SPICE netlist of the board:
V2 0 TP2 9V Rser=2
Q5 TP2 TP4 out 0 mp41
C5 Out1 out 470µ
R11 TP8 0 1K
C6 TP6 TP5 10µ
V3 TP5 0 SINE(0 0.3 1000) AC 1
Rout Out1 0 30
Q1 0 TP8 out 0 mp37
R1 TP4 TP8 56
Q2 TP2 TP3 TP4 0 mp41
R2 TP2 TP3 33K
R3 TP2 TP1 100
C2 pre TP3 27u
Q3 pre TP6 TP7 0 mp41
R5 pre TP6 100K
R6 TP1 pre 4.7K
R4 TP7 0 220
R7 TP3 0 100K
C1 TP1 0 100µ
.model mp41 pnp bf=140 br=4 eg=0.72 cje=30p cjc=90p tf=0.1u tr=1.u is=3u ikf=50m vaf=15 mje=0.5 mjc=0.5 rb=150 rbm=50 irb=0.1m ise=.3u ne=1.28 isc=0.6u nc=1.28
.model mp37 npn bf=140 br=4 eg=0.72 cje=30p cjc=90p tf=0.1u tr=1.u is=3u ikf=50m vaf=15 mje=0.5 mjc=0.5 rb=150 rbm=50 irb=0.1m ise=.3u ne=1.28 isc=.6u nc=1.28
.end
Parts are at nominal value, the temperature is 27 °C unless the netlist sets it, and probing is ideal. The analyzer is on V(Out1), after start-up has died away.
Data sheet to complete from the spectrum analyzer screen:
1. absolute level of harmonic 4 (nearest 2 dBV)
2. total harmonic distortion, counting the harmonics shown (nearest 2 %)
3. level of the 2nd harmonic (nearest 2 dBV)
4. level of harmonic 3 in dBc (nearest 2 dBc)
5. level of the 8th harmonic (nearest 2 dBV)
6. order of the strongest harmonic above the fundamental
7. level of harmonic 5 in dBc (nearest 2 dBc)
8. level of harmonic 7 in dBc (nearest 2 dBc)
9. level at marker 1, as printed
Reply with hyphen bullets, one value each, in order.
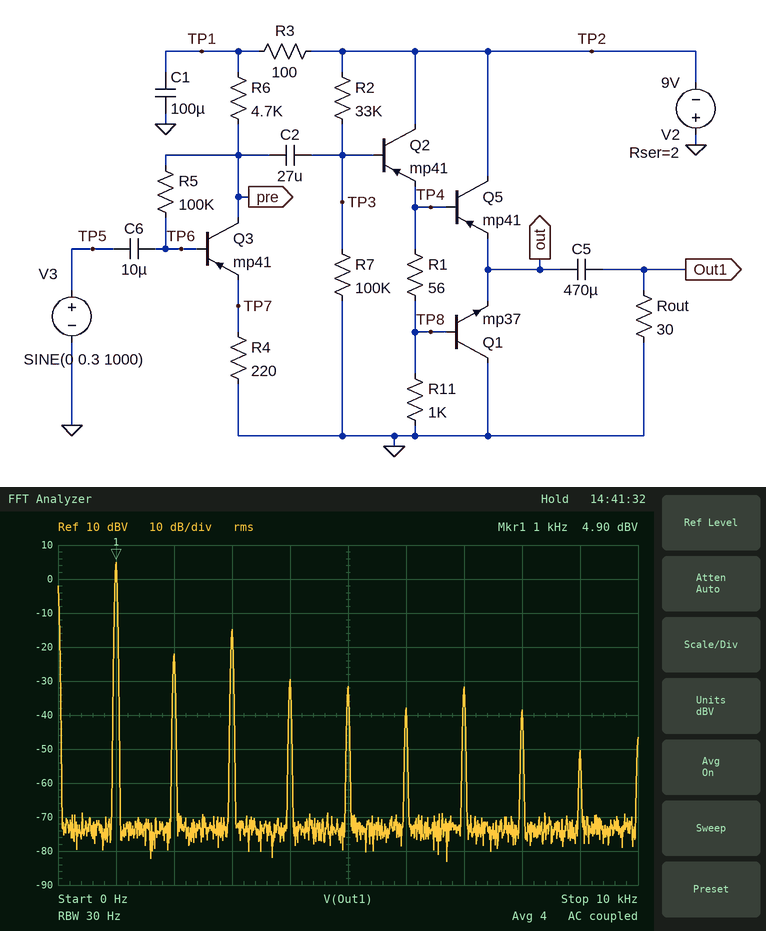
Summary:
- -30 dBV
- 12 %
- -22 dBV
- -20 dBc
- -38 dBV
- 3
- -36 dBc
- -36 dBc
- 4.90 dBV
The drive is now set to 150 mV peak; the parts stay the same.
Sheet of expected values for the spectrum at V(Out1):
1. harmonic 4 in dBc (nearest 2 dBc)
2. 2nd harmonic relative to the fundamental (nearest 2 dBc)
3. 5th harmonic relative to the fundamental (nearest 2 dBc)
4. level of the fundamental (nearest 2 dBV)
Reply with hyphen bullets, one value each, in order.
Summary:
- -52 dBc
- -48 dBc
- -40 dBc
- 0 dBV
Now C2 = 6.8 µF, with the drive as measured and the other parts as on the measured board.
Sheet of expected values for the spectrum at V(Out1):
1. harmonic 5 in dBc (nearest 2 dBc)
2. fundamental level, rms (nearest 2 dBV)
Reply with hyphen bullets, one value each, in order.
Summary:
- -40 dBc
- 4 dBV
